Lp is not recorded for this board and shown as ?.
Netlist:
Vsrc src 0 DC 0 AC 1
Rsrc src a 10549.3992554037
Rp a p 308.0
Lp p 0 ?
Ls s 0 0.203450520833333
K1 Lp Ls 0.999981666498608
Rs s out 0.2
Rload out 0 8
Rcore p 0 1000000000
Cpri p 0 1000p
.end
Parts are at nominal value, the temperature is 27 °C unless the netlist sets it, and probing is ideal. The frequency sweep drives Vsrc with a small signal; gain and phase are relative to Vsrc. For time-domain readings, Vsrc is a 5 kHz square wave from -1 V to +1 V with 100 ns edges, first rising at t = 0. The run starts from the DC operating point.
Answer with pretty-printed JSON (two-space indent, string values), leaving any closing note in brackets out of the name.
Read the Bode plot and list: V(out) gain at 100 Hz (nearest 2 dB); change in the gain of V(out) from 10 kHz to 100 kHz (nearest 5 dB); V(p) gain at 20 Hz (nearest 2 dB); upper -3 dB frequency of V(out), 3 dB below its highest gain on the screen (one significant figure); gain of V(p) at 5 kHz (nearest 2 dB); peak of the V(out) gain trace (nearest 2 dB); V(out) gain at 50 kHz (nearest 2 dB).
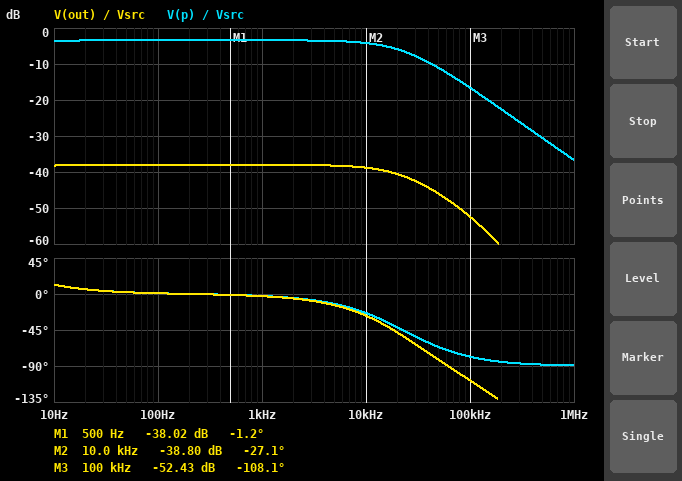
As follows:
{
  "V(out) gain at 100 Hz": "-38 dB",
  "change in the gain of V(out) from 10 kHz to 100 kHz": "-15 dB",
  "V(p) gain at 20 Hz": "-4 dB",
  "upper -3 dB frequency of V(out), 3 dB below its highest gain on the screen": "20 kHz",
  "gain of V(p) at 5 kHz": "-4 dB",
  "peak of the V(out) gain trace": "-38 dB",
  "V(out) gain at 50 kHz": "-46 dB"
}
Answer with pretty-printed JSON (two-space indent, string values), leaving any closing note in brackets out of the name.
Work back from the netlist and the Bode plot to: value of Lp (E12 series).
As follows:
{
  "value of Lp": "560 H"
}
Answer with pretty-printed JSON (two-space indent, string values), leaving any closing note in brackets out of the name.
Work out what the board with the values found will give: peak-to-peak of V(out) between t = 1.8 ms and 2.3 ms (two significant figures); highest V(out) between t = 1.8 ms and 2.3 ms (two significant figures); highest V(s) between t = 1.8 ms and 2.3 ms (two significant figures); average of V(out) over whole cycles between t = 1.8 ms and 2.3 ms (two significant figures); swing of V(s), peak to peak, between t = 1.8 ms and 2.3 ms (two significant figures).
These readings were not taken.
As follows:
{
  "peak-to-peak of V(out) between t = 1.8 ms and 2.3 ms": "25 mV",
  "highest V(out) between t = 1.8 ms and 2.3 ms": "25 mV",
  "highest V(s) between t = 1.8 ms and 2.3 ms": "25 mV",
  "average of V(out) over whole cycles between t = 1.8 ms and 2.3 ms": "12 mV",
  "swing of V(s), peak to peak, between t = 1.8 ms and 2.3 ms": "26 mV"
}
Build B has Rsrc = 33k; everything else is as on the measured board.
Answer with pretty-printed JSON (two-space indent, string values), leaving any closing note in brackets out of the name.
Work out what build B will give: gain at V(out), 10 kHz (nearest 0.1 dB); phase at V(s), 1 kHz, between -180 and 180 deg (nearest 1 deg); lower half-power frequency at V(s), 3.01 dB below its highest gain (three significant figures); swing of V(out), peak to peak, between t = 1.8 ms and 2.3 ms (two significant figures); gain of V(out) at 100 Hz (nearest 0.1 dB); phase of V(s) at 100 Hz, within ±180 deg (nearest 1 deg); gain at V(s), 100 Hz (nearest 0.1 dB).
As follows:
{
  "gain at V(out), 10 kHz": "-44.7 dB",
  "phase at V(s), 1 kHz, between -180 and 180 deg": "-5 deg",
  "lower half-power frequency at V(s), 3.01 dB below its highest gain": "3.82 Hz",
  "swing of V(out), peak to peak, between t = 1.8 ms and 2.3 ms": "15 mV",
  "gain of V(out) at 100 Hz": "-42.5 dB",
  "phase of V(s) at 100 Hz, within ±180 deg": "2 deg",
  "gain at V(s), 100 Hz": "-42.3 dB"
}
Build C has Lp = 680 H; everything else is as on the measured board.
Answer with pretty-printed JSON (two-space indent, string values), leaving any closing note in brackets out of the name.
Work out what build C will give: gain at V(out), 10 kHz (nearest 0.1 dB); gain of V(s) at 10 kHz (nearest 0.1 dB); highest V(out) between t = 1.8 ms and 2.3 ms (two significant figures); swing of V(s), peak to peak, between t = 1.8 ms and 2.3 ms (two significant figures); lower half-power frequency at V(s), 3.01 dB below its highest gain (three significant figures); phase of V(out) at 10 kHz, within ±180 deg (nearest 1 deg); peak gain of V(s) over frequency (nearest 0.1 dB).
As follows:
{
  "gain at V(out), 10 kHz": "-39.2 dB",
  "gain of V(s) at 10 kHz": "-39.0 dB",
  "highest V(out) between t = 1.8 ms and 2.3 ms": "24 mV",
  "swing of V(s), peak to peak, between t = 1.8 ms and 2.3 ms": "25 mV",
  "lower half-power frequency at V(s), 3.01 dB below its highest gain": "1.82 Hz",
  "phase of V(out) at 10 kHz, within ±180 deg": "-29 deg",
  "peak gain of V(s) over frequency": "-38.1 dB"
}
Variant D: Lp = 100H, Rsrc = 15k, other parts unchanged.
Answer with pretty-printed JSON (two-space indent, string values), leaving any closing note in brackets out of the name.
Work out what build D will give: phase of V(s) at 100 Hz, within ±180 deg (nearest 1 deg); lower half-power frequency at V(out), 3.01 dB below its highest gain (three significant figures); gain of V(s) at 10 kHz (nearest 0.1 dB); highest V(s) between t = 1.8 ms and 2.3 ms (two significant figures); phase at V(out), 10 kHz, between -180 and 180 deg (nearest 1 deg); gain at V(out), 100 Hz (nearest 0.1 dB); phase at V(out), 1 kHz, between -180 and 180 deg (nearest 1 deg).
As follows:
{
  "phase of V(s) at 100 Hz, within ±180 deg": "3 deg",
  "lower half-power frequency at V(out), 3.01 dB below its highest gain": "5.08 Hz",
  "gain of V(s) at 10 kHz": "-40.6 dB",
  "highest V(s) between t = 1.8 ms and 2.3 ms": "18 mV",
  "phase at V(out), 10 kHz, between -180 and 180 deg": "-12 deg",
  "gain at V(out), 100 Hz": "-40.8 dB",
  "phase at V(out), 1 kHz, between -180 and 180 deg": "-1 deg"
}
